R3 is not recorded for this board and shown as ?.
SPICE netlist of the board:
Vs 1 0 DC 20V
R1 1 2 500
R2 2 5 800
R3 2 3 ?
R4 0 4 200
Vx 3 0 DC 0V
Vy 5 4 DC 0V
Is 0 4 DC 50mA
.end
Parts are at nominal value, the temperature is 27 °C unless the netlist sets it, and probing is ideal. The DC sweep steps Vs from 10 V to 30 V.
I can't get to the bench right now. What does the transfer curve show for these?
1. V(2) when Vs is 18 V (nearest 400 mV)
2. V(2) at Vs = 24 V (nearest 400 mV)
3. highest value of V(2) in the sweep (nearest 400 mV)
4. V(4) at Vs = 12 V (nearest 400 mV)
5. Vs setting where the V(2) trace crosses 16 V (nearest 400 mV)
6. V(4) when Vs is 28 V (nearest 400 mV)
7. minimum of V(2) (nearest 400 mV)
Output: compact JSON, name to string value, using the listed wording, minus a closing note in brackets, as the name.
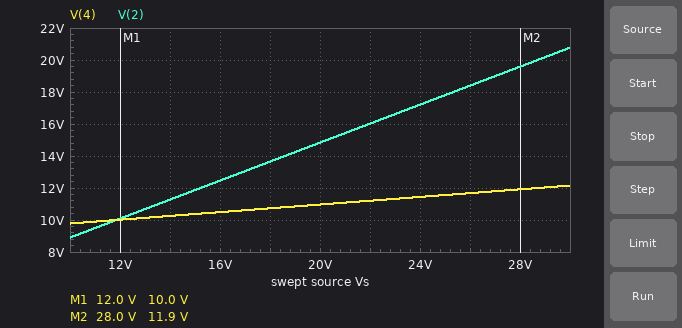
{"V(2) when Vs is 18 V": "13.6 V", "V(2) at Vs = 24 V": "17.2 V", "highest value of V(2) in the sweep": "20.8 V", "V(4) at Vs = 12 V": "10.0 V", "Vs setting where the V(2) trace crosses 16 V": "22.0 V", "V(4) when Vs is 28 V": "12.0 V", "minimum of V(2)": "8.8 V"}
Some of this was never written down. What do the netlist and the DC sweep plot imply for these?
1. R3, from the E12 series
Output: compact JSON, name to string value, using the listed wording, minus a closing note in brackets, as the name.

{"R3, from the E12 series": "2.7 kΩ"}
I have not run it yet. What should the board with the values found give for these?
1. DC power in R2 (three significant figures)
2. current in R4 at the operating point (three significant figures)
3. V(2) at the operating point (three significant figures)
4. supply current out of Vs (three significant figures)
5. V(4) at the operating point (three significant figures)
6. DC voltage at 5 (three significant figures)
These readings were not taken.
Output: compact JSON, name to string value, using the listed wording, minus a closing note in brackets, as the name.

{"DC power in R2": "18.7 mW", "current in R4 at the operating point": "54.8 mA", "V(2) at the operating point": "14.8 V", "supply current out of Vs": "10.3 mA", "V(4) at the operating point": "11.0 V", "DC voltage at 5": "11.0 V"}
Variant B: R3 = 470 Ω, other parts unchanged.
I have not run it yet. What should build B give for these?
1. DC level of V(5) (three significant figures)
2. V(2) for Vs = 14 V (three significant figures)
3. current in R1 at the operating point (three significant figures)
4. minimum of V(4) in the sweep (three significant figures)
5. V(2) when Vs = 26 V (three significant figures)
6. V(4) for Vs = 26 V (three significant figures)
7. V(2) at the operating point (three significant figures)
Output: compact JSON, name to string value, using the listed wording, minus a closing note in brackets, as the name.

{"DC level of V(5)": "9.95 V", "V(2) for Vs = 14 V": "7.41 V", "current in R1 at the operating point": "20.5 mA", "minimum of V(4) in the sweep": "9.17 V", "V(2) when Vs = 26 V": "12.1 V", "V(4) for Vs = 26 V": "10.4 V", "V(2) at the operating point": "9.75 V"}
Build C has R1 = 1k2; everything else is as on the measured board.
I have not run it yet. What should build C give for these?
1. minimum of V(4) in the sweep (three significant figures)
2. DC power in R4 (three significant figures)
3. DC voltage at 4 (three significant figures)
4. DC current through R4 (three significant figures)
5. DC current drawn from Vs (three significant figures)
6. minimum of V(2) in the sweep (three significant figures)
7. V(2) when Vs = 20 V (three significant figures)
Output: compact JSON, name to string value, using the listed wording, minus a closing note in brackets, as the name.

{"minimum of V(4) in the sweep": "9.66 V", "DC power in R4": "543 mW", "DC voltage at 4": "10.4 V", "DC current through R4": "52.1 mA", "DC current drawn from Vs": "6.58 mA", "minimum of V(2) in the sweep": "8.32 V", "V(2) when Vs = 20 V": "12.1 V"}
